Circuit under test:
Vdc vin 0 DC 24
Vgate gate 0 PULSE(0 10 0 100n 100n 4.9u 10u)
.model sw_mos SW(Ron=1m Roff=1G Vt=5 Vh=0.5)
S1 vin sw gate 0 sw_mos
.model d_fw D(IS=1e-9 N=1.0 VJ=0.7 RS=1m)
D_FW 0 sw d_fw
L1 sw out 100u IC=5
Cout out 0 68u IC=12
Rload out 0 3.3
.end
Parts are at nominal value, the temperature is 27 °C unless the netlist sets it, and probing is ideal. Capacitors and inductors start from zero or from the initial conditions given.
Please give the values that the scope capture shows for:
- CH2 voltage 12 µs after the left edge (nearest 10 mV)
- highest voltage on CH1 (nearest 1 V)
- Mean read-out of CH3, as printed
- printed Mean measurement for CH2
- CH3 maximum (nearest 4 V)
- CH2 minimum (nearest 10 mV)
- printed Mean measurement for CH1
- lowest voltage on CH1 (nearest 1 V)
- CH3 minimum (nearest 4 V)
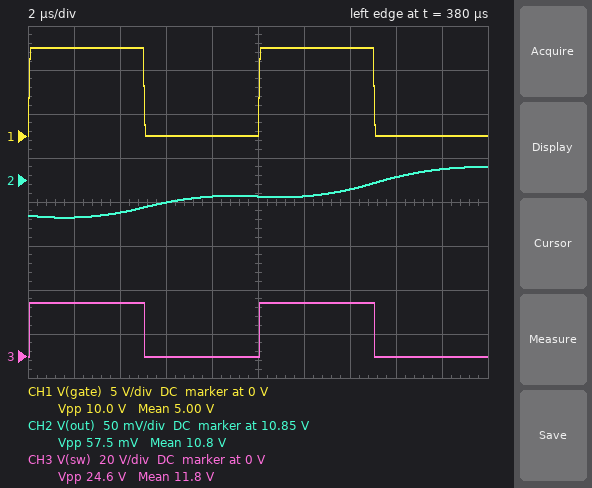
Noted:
10.83 V
10 V
11.8 V
10.8 V
24 V
10.81 V
5.00 V
0 V
0 V
